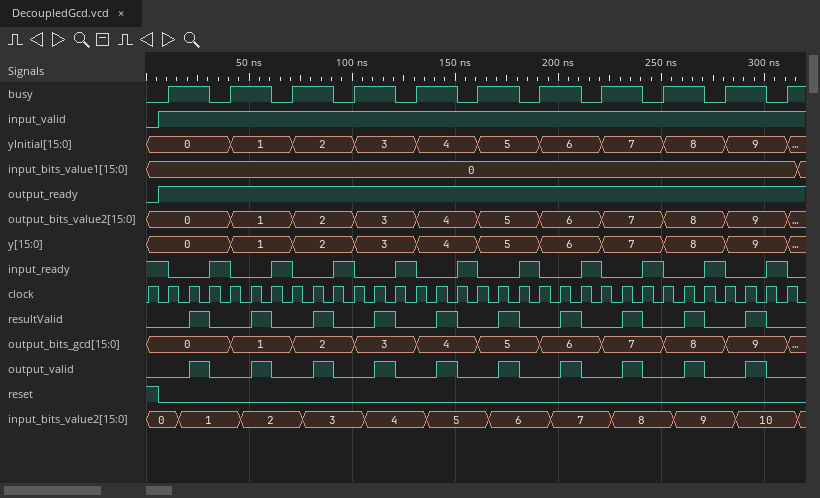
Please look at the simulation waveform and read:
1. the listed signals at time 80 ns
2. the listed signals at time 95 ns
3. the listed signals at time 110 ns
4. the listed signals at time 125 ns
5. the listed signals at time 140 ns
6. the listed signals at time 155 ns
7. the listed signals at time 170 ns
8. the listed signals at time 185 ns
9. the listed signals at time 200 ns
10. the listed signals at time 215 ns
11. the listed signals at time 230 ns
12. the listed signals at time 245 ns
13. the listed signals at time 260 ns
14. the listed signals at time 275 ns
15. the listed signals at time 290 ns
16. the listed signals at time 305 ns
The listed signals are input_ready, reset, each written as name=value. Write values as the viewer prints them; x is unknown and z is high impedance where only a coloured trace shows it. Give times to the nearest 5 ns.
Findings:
input_ready=0, reset=0
input_ready=1, reset=0
input_ready=0, reset=0
input_ready=1, reset=0
input_ready=0, reset=0
input_ready=1, reset=0
input_ready=0, reset=0
input_ready=1, reset=0
input_ready=0, reset=0
input_ready=1, reset=0
input_ready=0, reset=0
input_ready=1, reset=0
input_ready=0, reset=0
input_ready=1, reset=0
input_ready=0, reset=0
input_ready=1, reset=0
